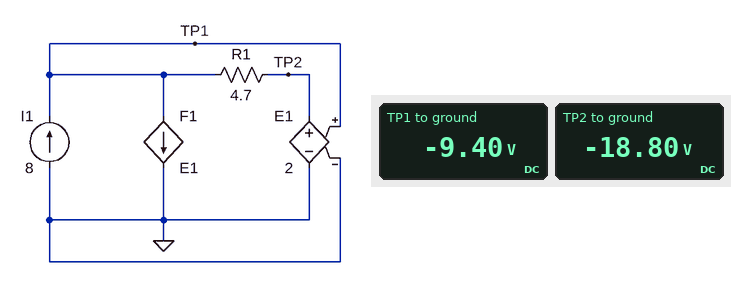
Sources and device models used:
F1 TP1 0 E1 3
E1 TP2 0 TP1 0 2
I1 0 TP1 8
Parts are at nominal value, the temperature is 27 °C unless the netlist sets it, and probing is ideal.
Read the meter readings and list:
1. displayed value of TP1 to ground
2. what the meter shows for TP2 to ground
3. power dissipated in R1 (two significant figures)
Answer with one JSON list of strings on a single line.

["-9.40 V", "-18.80 V", "19 W"]
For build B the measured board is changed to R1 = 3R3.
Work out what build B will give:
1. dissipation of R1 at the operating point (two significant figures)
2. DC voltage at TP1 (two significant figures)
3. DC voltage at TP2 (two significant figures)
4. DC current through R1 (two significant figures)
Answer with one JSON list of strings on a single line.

["13 W", "-6.6 V", "-13 V", "2.0 A"]
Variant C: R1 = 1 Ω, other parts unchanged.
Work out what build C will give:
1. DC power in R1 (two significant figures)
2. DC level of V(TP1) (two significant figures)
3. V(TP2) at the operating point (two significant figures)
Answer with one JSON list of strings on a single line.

["4.0 W", "-2.0 V", "-4.0 V"]
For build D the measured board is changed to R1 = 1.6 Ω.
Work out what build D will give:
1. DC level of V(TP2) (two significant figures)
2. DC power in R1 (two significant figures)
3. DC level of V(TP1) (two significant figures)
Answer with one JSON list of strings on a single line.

["-6.4 V", "6.4 W", "-3.2 V"]
